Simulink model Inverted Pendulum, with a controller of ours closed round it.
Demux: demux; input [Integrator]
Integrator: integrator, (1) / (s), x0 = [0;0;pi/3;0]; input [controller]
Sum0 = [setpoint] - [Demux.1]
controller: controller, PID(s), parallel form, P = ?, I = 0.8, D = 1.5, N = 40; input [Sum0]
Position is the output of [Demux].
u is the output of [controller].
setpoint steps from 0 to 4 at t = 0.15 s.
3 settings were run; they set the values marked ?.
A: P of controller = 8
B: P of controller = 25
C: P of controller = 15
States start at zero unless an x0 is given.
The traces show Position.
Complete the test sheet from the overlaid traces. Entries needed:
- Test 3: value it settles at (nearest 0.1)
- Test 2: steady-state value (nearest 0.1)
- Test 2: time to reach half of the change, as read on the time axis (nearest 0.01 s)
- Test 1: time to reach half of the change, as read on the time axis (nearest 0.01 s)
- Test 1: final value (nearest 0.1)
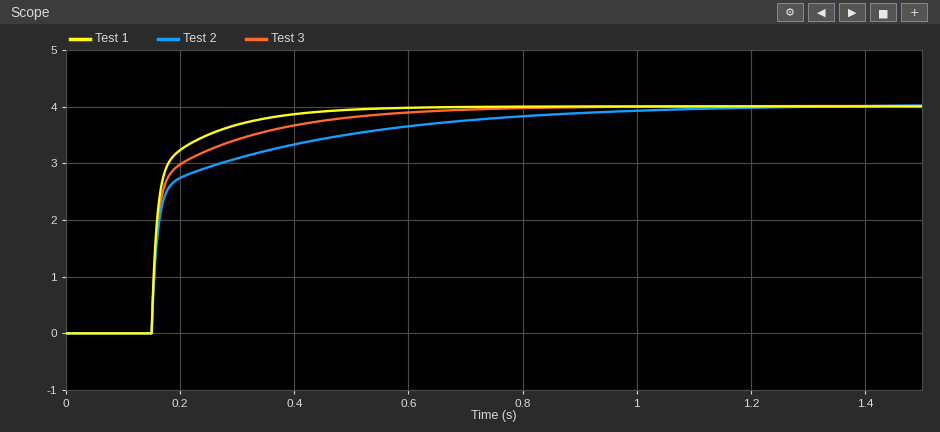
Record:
4.0
4.0
0.16 s
0.16 s
4.0
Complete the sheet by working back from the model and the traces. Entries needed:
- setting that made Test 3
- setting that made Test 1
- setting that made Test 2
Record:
C
B
A
